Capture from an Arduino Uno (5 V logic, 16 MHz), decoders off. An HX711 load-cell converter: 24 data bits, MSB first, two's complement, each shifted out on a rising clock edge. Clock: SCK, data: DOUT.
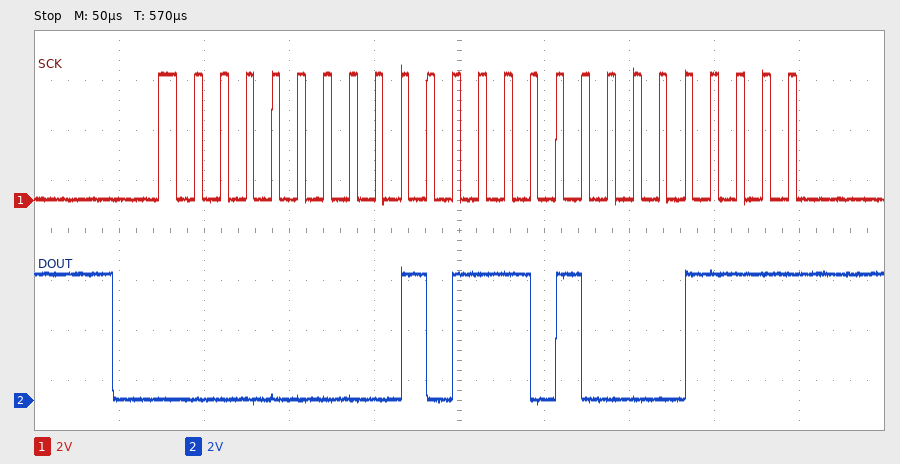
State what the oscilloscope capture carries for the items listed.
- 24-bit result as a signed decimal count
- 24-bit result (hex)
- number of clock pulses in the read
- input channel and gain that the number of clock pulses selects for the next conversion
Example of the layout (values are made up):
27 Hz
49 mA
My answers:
23823
0x005D0F
25
channel A, gain 128
